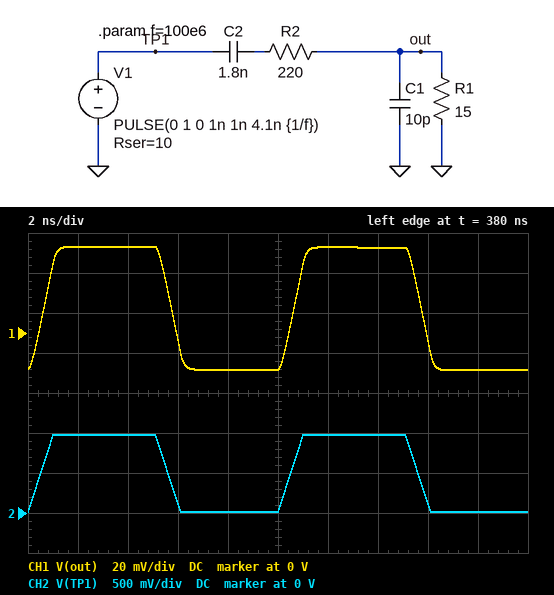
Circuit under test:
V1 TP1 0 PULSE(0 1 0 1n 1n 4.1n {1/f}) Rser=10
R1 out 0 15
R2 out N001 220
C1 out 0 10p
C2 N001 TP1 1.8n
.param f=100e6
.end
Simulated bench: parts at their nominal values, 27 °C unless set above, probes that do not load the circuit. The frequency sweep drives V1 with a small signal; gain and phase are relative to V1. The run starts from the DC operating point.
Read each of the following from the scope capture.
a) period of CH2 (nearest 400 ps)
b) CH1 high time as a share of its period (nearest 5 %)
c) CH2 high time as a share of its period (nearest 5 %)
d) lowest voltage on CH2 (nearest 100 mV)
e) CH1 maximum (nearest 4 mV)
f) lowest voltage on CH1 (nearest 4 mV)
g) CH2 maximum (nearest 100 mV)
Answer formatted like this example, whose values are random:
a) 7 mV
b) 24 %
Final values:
a) 10.0 ns
b) 50 %
c) 50 %
d) 0 V
e) 44 mV
f) -20 mV
g) 1.0 V
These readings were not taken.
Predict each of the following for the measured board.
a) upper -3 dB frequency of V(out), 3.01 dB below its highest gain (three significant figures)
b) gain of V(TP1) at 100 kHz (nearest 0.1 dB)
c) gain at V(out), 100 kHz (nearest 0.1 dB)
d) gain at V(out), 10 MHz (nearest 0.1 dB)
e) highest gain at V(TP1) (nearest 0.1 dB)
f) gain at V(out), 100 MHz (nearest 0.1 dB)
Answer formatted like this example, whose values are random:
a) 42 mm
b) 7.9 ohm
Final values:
a) 1.13 GHz
b) 0 dB
c) -35.7 dB
d) -24.3 dB
e) 0 dB
f) -24.3 dB
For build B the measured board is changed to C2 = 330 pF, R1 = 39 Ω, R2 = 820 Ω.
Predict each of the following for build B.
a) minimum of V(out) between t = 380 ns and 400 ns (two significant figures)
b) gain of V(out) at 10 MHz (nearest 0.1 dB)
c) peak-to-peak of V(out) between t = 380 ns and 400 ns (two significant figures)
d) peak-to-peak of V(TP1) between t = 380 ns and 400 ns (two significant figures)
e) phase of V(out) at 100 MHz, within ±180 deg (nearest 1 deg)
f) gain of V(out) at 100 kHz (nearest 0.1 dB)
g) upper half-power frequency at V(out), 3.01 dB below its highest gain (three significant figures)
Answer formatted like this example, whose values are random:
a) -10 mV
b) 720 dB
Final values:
a) -17 mV
b) -27.0 dB
c) 45 mV
d) 990 mV
e) -13 deg
f) -42.0 dB
g) 428 MHz
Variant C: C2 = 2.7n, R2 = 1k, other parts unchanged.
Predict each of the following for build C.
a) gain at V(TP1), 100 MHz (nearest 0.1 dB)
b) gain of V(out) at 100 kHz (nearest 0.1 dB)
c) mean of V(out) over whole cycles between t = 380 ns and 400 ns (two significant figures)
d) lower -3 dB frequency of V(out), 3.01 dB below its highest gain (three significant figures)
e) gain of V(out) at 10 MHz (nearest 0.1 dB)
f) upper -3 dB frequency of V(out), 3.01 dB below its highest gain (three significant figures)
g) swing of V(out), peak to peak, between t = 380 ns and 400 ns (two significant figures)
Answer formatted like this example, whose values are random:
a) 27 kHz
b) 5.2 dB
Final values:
a) -0.1 dB
b) -37.9 dB
c) 6.5 mV
d) 57.5 kHz
e) -36.7 dB
f) 1.08 GHz
g) 15 mV
